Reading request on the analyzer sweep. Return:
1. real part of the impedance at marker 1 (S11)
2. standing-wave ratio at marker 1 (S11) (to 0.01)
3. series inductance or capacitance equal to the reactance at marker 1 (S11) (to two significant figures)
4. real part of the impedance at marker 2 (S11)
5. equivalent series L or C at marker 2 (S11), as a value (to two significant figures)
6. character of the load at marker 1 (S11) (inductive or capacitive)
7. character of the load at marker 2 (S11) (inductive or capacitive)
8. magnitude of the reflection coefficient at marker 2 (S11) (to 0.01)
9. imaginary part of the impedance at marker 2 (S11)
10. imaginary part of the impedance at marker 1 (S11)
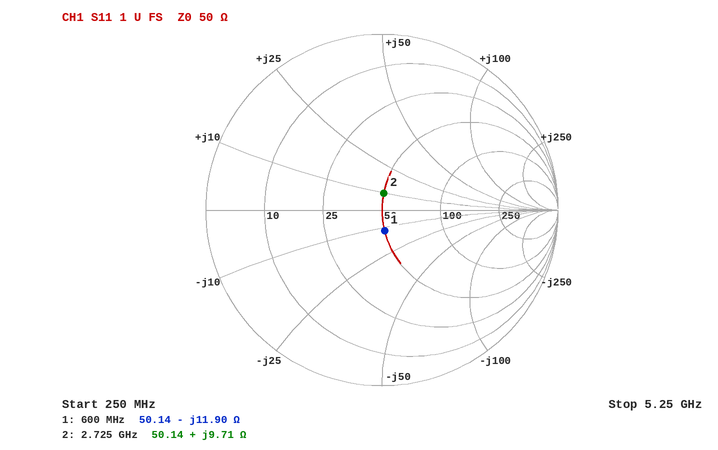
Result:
50.14 Ω
1.27
22 pF
50.14 Ω
570 pH
capacitive
inductive
0.10
+9.71 Ω
-11.90 Ω
